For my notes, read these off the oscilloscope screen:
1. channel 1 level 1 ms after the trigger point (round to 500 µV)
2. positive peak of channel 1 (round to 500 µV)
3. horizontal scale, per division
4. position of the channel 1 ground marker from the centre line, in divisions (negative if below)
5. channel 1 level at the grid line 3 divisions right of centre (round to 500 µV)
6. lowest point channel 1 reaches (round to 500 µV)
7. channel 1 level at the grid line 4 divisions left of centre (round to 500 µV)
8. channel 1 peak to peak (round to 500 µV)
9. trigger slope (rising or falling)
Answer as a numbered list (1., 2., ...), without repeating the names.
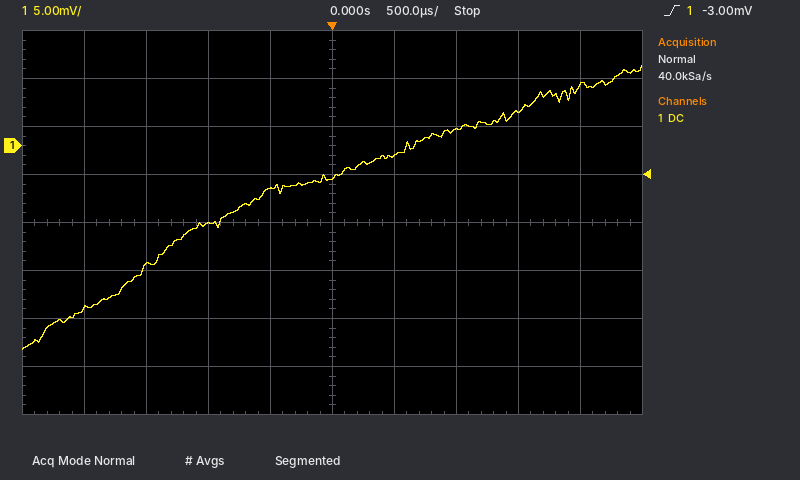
1. 1.5 mV
2. 8.5 mV
3. 500 µs
4. +1.6 div
5. 3.5 mV
6. -21.0 mV
7. -17.0 mV
8. 29.5 mV
9. rising
